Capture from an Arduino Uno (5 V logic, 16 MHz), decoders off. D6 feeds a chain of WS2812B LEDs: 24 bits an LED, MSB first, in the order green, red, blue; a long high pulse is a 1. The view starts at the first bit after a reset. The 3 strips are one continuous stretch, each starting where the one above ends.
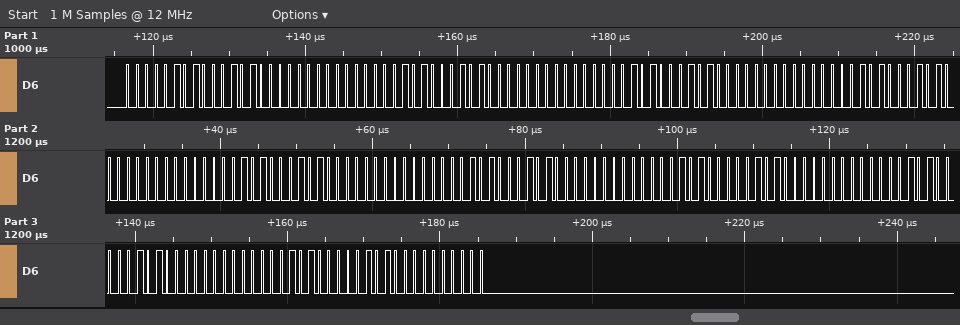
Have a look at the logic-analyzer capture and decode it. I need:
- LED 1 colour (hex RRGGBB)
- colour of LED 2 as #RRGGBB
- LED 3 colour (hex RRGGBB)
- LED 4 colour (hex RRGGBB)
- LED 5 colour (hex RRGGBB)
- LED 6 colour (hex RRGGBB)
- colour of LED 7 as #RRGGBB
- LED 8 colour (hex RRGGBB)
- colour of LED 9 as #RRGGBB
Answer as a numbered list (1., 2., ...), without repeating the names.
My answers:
1. #140500
2. #140500
3. #140500
4. #140500
5. #140500
6. #140500
7. #141400
8. #141400
9. #141400
